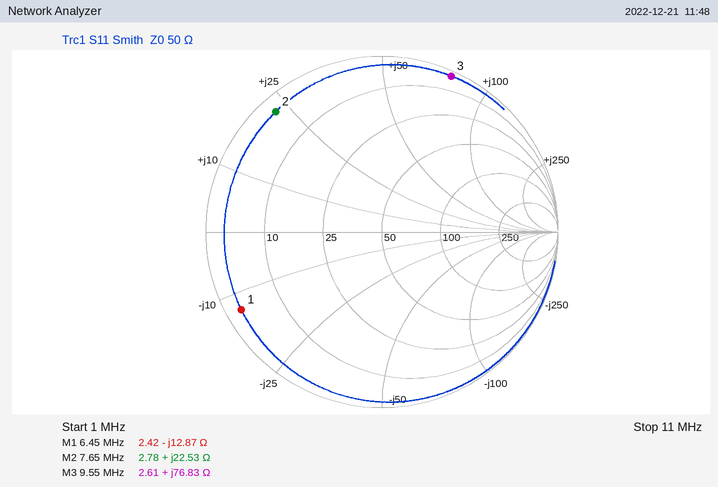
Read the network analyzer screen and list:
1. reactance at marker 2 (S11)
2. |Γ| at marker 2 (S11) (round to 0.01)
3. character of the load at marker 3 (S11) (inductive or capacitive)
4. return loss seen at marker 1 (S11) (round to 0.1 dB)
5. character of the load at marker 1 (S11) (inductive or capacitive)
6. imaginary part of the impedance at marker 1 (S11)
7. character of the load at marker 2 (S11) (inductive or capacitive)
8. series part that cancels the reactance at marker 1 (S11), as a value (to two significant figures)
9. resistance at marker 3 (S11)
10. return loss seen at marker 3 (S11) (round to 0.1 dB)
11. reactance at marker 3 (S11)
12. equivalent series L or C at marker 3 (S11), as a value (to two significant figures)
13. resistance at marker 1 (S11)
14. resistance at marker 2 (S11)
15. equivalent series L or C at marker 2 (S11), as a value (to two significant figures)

+22.53 Ω
0.91
inductive
0.8 dB
capacitive
-12.87 Ω
inductive
320 nH
2.61 Ω
0.3 dB
+76.83 Ω
1.3 µH
2.42 Ω
2.78 Ω
470 nH
